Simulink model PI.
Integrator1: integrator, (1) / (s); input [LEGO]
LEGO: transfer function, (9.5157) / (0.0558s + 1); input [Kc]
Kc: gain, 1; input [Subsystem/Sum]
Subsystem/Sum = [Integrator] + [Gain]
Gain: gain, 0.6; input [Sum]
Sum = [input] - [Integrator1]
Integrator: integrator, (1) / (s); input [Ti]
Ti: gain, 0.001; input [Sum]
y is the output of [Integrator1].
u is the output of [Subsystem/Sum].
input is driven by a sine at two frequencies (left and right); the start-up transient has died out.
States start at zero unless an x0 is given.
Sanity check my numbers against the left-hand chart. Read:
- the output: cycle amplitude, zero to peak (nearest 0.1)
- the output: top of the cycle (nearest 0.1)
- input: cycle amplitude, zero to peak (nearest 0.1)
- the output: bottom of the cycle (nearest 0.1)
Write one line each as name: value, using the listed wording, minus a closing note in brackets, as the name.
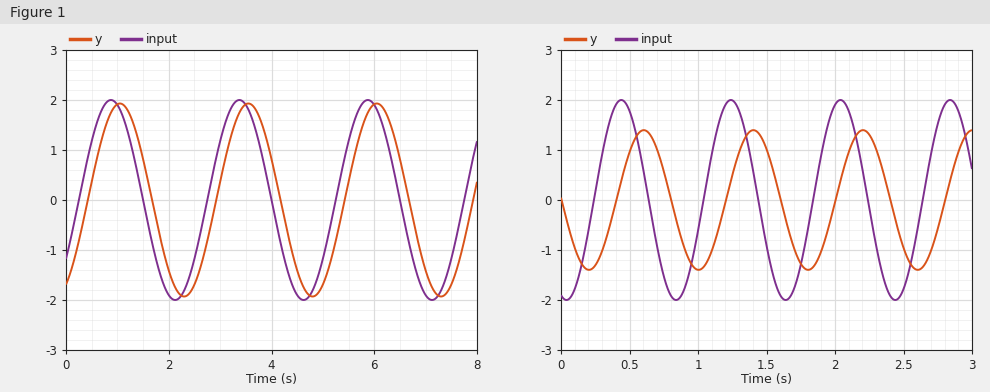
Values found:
the output: cycle amplitude, zero to peak: 1.9
the output: top of the cycle: 1.9
input: cycle amplitude, zero to peak: 2.0
the output: bottom of the cycle: -1.9
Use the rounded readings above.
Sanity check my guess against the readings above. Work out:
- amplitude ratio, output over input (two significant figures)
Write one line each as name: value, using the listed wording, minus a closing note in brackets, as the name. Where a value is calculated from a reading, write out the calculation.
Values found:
amplitude ratio, output over input: 1.9 / 2 = 0.95
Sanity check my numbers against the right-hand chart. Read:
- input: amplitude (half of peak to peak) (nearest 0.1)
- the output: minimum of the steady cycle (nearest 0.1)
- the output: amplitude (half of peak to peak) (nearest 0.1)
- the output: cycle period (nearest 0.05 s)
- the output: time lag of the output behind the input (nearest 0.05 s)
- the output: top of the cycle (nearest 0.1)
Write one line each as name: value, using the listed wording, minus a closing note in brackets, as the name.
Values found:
input: amplitude (half of peak to peak): 2.0
the output: minimum of the steady cycle: -1.4
the output: amplitude (half of peak to peak): 1.4
the output: cycle period: 0.80 s
the output: time lag of the output behind the input: 0.15 s
the output: top of the cycle: 1.4
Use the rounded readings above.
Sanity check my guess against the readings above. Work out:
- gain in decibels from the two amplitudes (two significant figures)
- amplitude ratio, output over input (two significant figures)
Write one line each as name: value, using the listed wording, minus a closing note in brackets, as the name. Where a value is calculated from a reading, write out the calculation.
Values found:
gain in decibels from the two amplitudes: 20 log10(1.4 / 2) = -3.1 dB
amplitude ratio, output over input: 1.4 / 2 = 0.70
